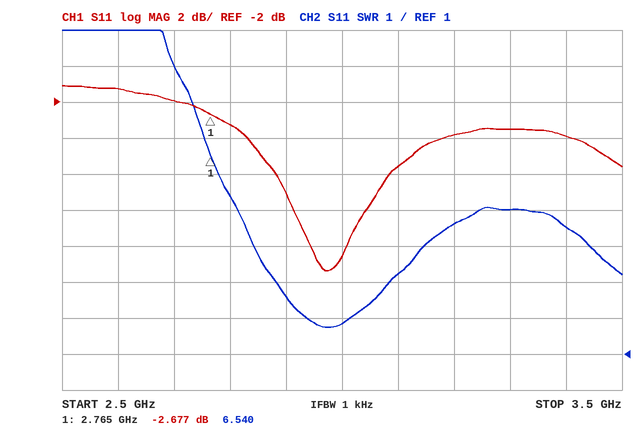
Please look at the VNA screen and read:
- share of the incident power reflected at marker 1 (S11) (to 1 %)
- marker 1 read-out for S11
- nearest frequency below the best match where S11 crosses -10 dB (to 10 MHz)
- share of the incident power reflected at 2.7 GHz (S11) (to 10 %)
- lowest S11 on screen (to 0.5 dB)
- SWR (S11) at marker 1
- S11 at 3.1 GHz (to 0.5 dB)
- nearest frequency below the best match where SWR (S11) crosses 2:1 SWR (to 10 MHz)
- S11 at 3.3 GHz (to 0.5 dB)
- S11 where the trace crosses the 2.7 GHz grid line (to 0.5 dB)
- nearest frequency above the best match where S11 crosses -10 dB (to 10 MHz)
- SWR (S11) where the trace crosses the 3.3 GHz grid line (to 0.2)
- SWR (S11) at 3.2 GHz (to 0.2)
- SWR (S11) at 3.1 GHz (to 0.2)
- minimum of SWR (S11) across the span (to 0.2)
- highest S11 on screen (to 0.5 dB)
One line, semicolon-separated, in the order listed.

54 %; -2.677 dB; 2.94 GHz; 60 %; -11.5 dB; 6.540; -5.5 dB; 2.94 GHz; -3.5 dB; -2.0 dB; 3.01 GHz; 5.0; 4.6; 3.2; 1.8; -1.0 dB
